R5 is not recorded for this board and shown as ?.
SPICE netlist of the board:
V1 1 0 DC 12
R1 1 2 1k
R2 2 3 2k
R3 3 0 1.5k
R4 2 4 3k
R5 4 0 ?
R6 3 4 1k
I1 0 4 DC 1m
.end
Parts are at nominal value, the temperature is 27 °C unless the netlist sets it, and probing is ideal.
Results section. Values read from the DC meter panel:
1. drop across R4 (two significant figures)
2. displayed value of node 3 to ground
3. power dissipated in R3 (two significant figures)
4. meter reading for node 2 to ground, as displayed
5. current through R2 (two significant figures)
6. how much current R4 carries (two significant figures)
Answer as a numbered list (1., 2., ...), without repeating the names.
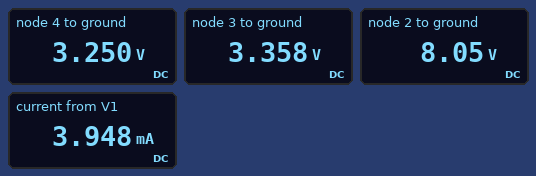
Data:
1. 4.8 V
2. 3.358 V
3. 7.5 mW
4. 8.05 V
5. 2.3 mA
6. 1.6 mA
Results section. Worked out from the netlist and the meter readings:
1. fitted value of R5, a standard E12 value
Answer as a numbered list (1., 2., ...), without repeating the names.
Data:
1. 1.2 kΩ
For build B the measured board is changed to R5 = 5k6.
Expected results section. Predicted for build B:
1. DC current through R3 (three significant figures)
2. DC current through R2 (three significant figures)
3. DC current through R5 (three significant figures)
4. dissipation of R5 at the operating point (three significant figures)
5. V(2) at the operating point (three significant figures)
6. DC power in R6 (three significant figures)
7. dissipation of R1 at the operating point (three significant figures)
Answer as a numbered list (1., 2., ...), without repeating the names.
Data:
1. 3.12 mA
2. 2.09 mA
3. 1.02 mA
4. 5.82 mW
5. 8.86 V
6. 1.06 mW
7. 9.86 mW
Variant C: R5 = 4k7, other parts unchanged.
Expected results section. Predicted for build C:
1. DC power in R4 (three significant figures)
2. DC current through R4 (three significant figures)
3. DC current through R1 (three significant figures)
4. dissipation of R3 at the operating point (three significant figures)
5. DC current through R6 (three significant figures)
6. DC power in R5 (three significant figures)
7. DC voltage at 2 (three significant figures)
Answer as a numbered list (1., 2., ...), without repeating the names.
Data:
1. 3.62 mW
2. 1.10 mA
3. 3.21 mA
4. 13.9 mW
5. 930 µA
6. 6.42 mW
7. 8.79 V
